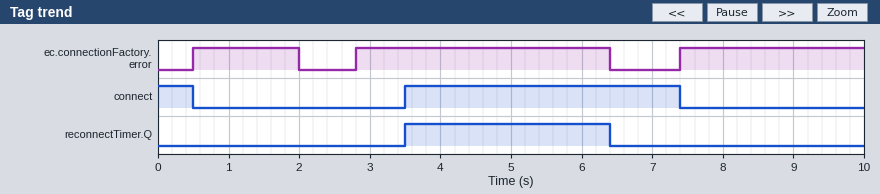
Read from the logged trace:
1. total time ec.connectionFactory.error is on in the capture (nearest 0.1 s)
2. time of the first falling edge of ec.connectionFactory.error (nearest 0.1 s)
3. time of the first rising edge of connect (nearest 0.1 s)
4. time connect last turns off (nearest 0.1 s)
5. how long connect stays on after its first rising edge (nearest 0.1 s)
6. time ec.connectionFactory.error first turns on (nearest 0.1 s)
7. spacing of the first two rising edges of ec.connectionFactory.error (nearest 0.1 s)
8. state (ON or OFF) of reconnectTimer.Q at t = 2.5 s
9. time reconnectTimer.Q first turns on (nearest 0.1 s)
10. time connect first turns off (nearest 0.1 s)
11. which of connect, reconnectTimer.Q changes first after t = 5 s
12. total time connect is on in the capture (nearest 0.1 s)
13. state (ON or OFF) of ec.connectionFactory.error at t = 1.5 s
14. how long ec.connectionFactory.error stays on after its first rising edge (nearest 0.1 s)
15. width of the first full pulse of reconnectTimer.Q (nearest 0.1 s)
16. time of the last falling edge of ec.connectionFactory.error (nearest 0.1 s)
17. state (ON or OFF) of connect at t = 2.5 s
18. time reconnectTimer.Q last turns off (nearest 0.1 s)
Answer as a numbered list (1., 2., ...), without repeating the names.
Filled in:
1. 7.7 s
2. 2.0 s
3. 3.5 s
4. 7.4 s
5. 3.9 s
6. 0.5 s
7. 2.3 s
8. OFF
9. 3.5 s
10. 0.5 s
11. reconnectTimer.Q
12. 4.4 s
13. ON
14. 1.5 s
15. 2.9 s
16. 6.4 s
17. OFF
18. 6.4 s
